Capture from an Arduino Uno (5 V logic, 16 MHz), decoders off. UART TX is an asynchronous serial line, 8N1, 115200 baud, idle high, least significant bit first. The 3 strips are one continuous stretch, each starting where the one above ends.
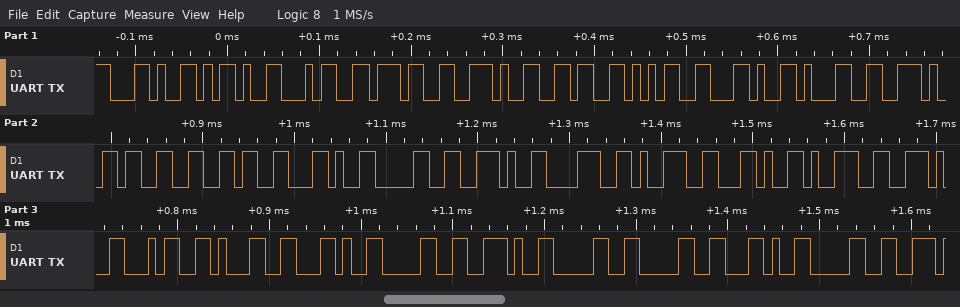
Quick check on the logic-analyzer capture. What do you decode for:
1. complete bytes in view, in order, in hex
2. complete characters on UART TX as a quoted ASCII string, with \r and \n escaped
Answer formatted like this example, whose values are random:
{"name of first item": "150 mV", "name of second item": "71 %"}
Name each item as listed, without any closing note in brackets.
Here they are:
{"complete bytes in view, in order, in hex": "2C 2D 34 37 2E 36 35 2C 31 2E 33 36 2C 30 2E 38 39 2C 39 2E 34 31 2C 30 2E 30 30 2C 30", "complete characters on UART TX as a quoted ASCII string, with \\r and \\n escaped": "\",-47.65,1.36,0.89,9.41,0.00,0\""}
